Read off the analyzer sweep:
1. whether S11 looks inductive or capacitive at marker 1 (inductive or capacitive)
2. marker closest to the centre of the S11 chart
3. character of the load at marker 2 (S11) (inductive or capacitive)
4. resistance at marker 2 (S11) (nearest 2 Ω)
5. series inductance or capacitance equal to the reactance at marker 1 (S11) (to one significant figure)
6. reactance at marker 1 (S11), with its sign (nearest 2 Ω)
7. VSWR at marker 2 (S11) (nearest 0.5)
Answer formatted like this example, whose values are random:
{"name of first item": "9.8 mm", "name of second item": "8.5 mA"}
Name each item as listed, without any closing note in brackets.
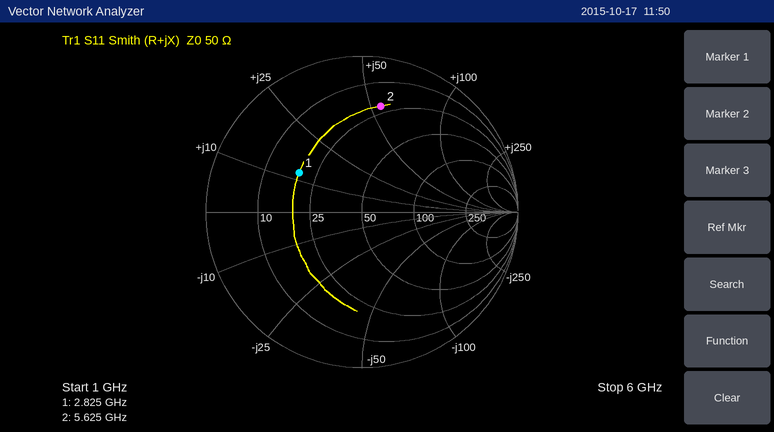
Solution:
{"whether S11 looks inductive or capacitive at marker 1": "inductive", "marker closest to the centre of the S11 chart": "marker 1", "character of the load at marker 2 (S11)": "inductive", "resistance at marker 2 (S11)": "22 Ω", "series inductance or capacitance equal to the reactance at marker 1 (S11)": "700 pH", "reactance at marker 1 (S11), with its sign": "+12 Ω", "VSWR at marker 2 (S11)": "5.5"}
